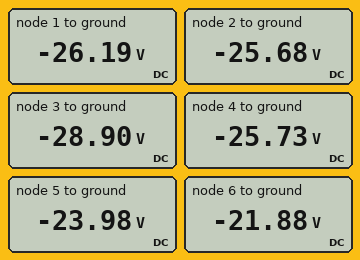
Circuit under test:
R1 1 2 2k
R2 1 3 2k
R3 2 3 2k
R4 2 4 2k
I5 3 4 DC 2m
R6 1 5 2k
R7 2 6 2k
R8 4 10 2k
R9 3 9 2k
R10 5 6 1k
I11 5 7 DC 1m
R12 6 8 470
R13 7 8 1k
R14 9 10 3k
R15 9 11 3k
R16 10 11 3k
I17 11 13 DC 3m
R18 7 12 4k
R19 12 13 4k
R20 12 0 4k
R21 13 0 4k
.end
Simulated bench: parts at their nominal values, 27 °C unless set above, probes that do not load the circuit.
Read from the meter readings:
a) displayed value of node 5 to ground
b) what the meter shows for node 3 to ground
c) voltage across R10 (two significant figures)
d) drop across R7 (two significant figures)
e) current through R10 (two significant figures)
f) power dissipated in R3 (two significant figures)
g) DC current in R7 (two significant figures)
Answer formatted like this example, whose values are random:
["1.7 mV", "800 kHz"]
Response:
["-23.98 V", "-28.90 V", "2.1 V", "3.8 V", "2.1 mA", "5.2 mW", "1.9 mA"]
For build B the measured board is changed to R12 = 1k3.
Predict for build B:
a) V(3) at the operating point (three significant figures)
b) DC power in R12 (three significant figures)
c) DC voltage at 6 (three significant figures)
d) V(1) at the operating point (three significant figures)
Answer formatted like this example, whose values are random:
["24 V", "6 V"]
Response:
["-32.2 V", "20.8 mW", "-25.2 V", "-29.5 V"]
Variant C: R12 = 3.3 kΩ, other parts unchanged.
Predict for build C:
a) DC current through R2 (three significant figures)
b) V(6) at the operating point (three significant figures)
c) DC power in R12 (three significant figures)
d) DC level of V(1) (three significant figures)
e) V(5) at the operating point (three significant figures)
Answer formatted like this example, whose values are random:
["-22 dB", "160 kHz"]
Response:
["1.36 mA", "-33.2 V", "52.8 mW", "-37.5 V", "-35.3 V"]
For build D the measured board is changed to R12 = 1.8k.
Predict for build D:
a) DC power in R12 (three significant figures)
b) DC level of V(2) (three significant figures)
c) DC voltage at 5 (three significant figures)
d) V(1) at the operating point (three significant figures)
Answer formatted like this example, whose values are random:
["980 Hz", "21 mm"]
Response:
["28.8 mW", "-31.0 V", "-29.3 V", "-31.5 V"]
